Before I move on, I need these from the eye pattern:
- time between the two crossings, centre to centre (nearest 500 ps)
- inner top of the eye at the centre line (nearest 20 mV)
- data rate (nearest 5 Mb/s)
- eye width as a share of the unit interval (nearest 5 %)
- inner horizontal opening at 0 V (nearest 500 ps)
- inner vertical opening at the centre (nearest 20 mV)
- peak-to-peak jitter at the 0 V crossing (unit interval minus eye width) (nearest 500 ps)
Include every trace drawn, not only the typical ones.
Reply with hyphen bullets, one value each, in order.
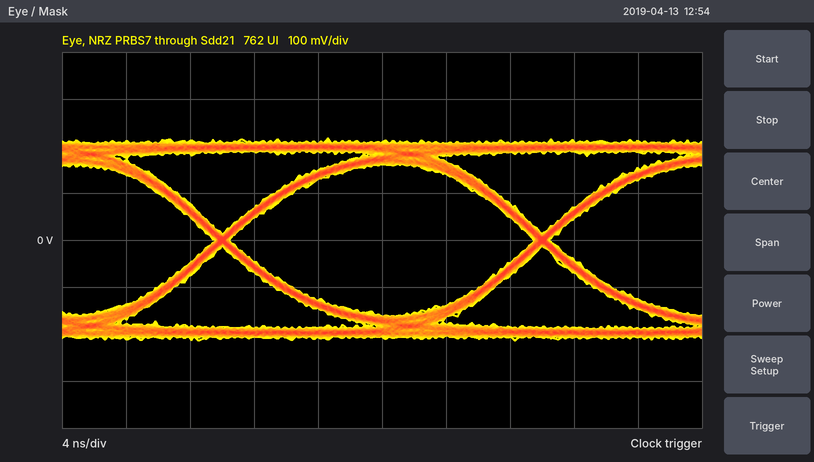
- 20.0 ns
- 160 mV
- 50 Mb/s
- 95 %
- 19.0 ns
- 320 mV
- 1.0 ns
